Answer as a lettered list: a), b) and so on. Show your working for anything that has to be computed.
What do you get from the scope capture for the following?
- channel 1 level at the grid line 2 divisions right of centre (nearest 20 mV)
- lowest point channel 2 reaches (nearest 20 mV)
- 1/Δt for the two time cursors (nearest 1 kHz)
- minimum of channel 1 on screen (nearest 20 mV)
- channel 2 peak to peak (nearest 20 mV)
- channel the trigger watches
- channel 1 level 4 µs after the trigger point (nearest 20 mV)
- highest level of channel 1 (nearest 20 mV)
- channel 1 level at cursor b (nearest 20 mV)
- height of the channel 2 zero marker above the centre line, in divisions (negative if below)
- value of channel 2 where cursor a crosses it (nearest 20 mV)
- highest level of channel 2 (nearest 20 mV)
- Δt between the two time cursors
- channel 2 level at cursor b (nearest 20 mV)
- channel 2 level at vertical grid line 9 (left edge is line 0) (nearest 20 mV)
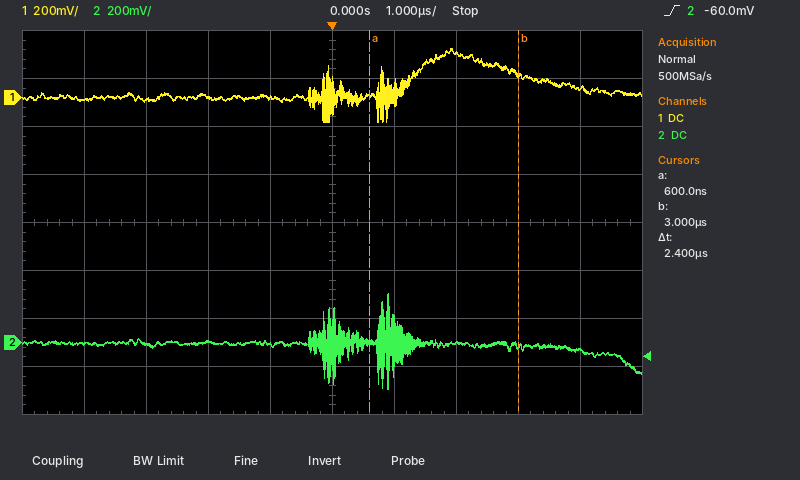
a) 180 mV
b) -200 mV
c) 1 / 2.4 µs ≈ 417 kHz
d) -100 mV
e) 200 mV − (-200 mV) = 400 mV
f) channel 2
g) 40 mV
h) 200 mV
i) 100 mV
j) -2.5 div
k) 0 mV
l) 200 mV
m) 2.4 µs
n) -20 mV
o) -40 mV
